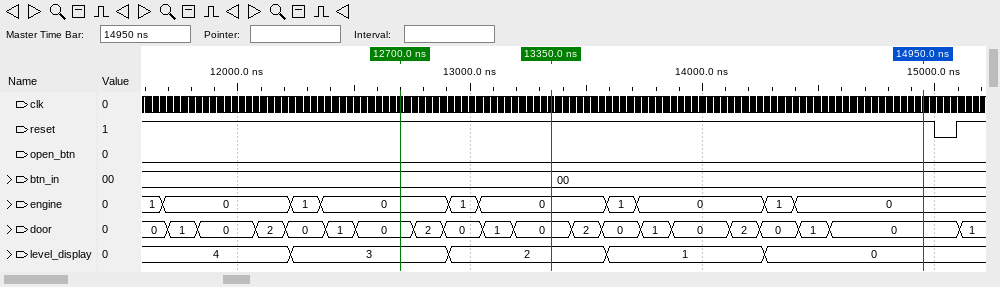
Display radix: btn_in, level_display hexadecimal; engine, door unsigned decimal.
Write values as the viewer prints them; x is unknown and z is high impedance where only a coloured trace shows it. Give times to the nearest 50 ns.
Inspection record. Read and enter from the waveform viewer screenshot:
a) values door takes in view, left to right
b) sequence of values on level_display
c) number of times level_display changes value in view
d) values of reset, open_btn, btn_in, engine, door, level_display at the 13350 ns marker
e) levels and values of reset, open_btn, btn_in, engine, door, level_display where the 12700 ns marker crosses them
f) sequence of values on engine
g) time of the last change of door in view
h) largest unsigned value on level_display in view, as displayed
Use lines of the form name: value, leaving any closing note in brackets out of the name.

values door takes in view, left to right: 0, 1, 0, 2, 0, 1, 0, 2, 0, 1, 0, 2, 0, 1, 0, 2, 0, 1, 0, 1
sequence of values on level_display: 4, 3, 2, 1, 0
number of times level_display changes value in view: 4
values of reset, open_btn, btn_in, engine, door, level_display at the 13350 ns marker: reset=1, open_btn=0, btn_in=00, engine=0, door=0, level_display=2
levels and values of reset, open_btn, btn_in, engine, door, level_display where the 12700 ns marker crosses them: reset=1, open_btn=0, btn_in=00, engine=0, door=0, level_display=3
sequence of values on engine: 1, 0, 1, 0, 1, 0, 1, 0, 1, 0
time of the last change of door in view: 15100 ns
largest unsigned value on level_display in view, as displayed: 4
